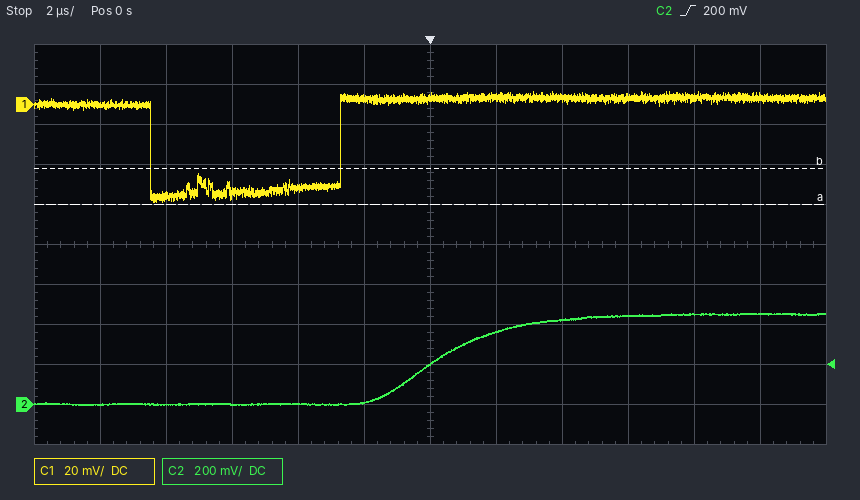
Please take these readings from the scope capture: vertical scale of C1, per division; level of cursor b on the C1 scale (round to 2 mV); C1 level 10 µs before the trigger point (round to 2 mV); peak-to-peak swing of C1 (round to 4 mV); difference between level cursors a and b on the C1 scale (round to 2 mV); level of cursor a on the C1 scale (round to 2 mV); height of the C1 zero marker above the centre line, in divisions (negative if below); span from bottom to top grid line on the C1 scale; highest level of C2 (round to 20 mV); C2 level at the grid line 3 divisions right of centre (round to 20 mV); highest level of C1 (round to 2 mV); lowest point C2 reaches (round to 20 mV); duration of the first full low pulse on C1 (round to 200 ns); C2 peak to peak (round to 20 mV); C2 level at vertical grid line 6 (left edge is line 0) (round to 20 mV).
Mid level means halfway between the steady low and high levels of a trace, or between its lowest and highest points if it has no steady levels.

20 mV
-32 mV
0 mV
56 mV
18 mV
-50 mV
+3.5 div
200 mV
460 mV
440 mV
6 mV
0 mV
5.8 µs
460 mV
200 mV
